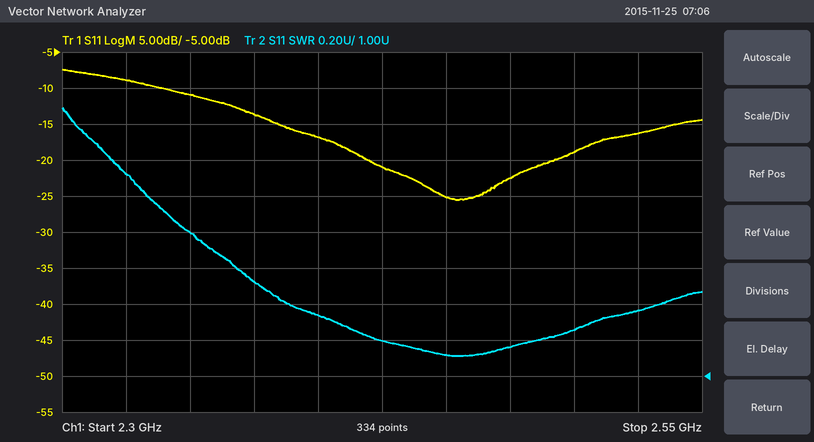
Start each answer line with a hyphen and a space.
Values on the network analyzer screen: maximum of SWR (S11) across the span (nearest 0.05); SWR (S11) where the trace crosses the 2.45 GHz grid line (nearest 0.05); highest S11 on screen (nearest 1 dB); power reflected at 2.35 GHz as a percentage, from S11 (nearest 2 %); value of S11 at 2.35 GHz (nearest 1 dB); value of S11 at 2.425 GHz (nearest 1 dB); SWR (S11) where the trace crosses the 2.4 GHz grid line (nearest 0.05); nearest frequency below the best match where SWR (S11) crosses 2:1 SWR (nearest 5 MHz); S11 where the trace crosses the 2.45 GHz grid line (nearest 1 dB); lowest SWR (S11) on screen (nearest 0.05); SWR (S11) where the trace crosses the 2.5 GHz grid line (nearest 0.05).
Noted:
- 2.50
- 1.10
- -7 dB
- 8 %
- -11 dB
- -21 dB
- 1.35
- 2.335 GHz
- -25 dB
- 1.10
- 1.25
